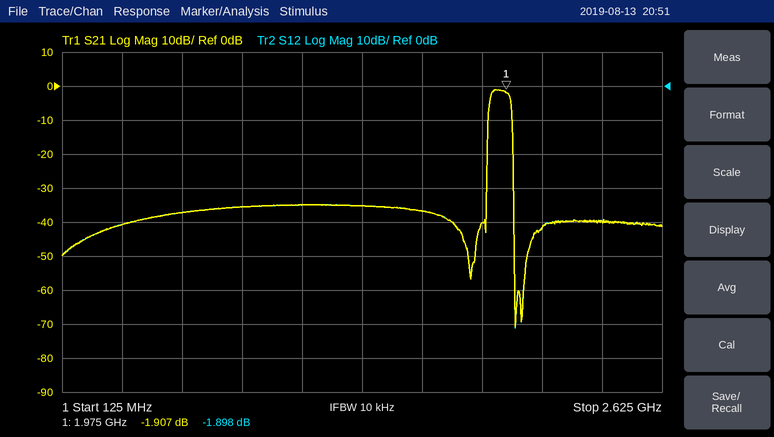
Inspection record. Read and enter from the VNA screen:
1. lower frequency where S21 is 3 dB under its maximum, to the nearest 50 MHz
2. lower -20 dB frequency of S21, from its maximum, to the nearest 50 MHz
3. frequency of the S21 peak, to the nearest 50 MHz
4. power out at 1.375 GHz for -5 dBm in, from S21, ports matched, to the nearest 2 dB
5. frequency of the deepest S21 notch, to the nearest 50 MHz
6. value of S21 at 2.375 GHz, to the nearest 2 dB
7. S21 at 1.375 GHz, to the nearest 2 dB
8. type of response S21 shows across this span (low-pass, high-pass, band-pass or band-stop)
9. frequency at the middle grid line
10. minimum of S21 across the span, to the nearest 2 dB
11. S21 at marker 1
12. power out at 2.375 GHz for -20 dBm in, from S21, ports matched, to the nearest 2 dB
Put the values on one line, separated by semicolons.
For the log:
1.90 GHz; 1.90 GHz; 1.95 GHz; -40 dBm; 2.00 GHz; -40 dB; -36 dB; band-pass; 1.375 GHz; -70 dB; -1.907 dB; -60 dBm
